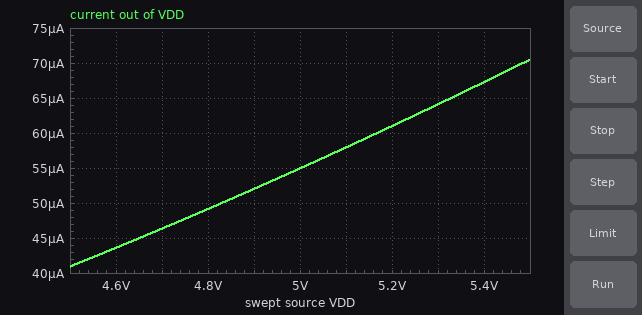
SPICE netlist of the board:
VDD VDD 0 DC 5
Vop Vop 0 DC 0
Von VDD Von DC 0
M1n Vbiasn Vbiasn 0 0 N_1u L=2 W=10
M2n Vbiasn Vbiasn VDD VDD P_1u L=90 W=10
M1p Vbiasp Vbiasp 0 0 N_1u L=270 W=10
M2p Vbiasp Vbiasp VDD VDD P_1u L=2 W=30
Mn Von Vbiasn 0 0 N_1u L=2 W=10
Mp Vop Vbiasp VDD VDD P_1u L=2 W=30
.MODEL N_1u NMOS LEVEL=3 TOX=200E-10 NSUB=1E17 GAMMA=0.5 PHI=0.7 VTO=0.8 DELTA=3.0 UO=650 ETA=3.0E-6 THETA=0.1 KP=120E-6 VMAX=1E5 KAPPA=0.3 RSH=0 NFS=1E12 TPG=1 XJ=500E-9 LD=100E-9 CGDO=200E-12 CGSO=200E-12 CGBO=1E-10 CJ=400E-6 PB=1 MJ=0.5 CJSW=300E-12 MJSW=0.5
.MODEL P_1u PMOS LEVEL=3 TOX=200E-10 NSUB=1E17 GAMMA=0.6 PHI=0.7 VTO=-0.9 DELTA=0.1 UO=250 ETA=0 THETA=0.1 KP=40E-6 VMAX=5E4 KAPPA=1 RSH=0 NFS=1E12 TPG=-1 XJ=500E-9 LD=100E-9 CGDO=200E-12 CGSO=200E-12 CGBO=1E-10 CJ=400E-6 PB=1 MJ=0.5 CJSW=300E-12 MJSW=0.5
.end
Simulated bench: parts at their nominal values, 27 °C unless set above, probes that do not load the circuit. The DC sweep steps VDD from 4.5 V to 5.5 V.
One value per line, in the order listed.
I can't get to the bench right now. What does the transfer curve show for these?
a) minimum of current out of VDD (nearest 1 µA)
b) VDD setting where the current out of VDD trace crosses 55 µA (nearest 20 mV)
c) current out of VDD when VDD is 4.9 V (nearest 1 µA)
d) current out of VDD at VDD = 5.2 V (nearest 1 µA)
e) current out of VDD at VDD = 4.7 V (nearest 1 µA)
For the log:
41 µA
5.00 V
52 µA
61 µA
46 µA
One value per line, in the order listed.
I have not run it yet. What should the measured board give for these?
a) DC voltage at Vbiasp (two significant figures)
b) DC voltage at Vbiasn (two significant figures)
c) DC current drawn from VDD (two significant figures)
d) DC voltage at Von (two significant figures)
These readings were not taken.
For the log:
3.9 V
1.0 V
55 µA
5.0 V
